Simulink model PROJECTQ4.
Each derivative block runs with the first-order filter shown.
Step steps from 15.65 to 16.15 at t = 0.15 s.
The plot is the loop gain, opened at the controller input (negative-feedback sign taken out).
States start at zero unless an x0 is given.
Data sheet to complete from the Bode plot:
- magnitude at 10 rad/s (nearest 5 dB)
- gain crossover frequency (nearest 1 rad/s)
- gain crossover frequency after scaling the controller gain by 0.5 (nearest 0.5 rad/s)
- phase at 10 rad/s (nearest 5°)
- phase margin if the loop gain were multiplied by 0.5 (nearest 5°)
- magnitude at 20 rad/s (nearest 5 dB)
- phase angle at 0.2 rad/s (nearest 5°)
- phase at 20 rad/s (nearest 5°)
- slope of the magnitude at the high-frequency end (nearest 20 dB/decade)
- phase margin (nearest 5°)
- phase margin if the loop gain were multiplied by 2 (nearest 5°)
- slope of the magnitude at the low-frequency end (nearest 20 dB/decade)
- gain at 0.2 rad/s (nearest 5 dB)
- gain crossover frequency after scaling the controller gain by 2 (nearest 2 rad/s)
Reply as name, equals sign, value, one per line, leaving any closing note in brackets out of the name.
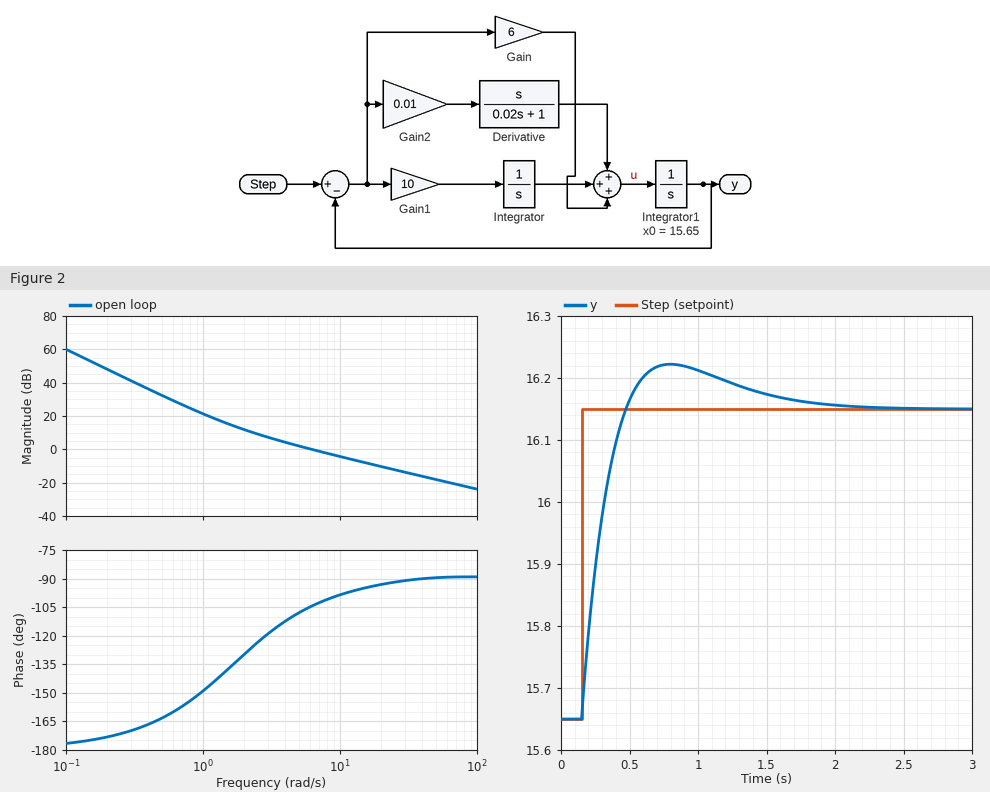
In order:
magnitude at 10 rad/s = -5 dB
gain crossover frequency = 6 rad/s
gain crossover frequency after scaling the controller gain by 0.5 = 3.5 rad/s
phase at 10 rad/s = -100°
phase margin if the loop gain were multiplied by 0.5 = 65°
magnitude at 20 rad/s = -10 dB
phase angle at 0.2 rad/s = -175°
phase at 20 rad/s = -95°
slope of the magnitude at the high-frequency end = -20 dB/decade
phase margin = 75°
phase margin if the loop gain were multiplied by 2 = 85°
slope of the magnitude at the low-frequency end = -40 dB/decade
gain at 0.2 rad/s = 50 dB
gain crossover frequency after scaling the controller gain by 2 = 12 rad/s
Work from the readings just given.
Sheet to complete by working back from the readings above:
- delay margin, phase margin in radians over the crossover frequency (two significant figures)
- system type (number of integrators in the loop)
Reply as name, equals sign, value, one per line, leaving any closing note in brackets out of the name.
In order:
delay margin, phase margin in radians over the crossover frequency = 0.22 s
system type = 2
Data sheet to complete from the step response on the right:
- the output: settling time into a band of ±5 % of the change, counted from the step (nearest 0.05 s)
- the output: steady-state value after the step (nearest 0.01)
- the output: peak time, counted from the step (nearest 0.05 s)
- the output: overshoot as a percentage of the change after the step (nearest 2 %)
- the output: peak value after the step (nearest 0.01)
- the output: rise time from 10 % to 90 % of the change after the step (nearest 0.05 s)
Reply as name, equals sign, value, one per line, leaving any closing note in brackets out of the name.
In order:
the output: settling time into a band of ±5 % of the change, counted from the step = 1.35 s
the output: steady-state value after the step = 16.15
the output: peak time, counted from the step = 0.65 s
the output: overshoot as a percentage of the change after the step = 14 %
the output: peak value after the step = 16.22
the output: rise time from 10 % to 90 % of the change after the step = 0.25 s
